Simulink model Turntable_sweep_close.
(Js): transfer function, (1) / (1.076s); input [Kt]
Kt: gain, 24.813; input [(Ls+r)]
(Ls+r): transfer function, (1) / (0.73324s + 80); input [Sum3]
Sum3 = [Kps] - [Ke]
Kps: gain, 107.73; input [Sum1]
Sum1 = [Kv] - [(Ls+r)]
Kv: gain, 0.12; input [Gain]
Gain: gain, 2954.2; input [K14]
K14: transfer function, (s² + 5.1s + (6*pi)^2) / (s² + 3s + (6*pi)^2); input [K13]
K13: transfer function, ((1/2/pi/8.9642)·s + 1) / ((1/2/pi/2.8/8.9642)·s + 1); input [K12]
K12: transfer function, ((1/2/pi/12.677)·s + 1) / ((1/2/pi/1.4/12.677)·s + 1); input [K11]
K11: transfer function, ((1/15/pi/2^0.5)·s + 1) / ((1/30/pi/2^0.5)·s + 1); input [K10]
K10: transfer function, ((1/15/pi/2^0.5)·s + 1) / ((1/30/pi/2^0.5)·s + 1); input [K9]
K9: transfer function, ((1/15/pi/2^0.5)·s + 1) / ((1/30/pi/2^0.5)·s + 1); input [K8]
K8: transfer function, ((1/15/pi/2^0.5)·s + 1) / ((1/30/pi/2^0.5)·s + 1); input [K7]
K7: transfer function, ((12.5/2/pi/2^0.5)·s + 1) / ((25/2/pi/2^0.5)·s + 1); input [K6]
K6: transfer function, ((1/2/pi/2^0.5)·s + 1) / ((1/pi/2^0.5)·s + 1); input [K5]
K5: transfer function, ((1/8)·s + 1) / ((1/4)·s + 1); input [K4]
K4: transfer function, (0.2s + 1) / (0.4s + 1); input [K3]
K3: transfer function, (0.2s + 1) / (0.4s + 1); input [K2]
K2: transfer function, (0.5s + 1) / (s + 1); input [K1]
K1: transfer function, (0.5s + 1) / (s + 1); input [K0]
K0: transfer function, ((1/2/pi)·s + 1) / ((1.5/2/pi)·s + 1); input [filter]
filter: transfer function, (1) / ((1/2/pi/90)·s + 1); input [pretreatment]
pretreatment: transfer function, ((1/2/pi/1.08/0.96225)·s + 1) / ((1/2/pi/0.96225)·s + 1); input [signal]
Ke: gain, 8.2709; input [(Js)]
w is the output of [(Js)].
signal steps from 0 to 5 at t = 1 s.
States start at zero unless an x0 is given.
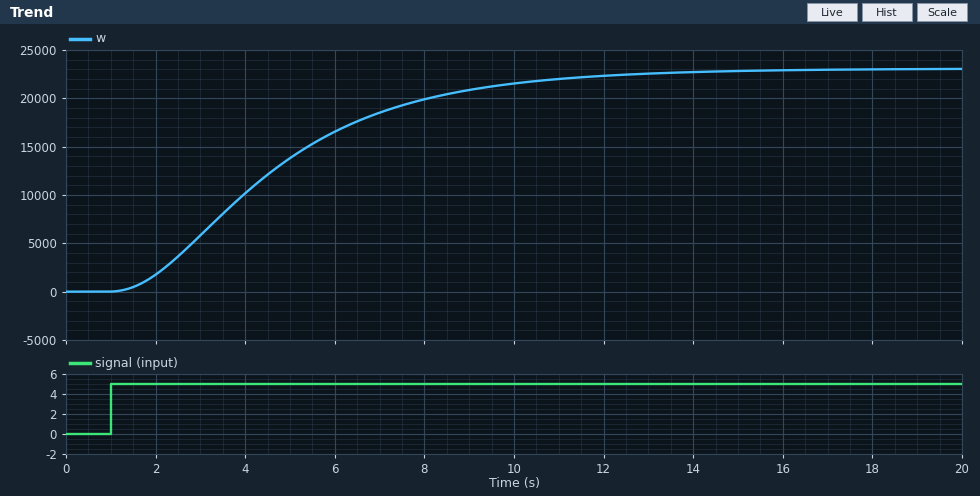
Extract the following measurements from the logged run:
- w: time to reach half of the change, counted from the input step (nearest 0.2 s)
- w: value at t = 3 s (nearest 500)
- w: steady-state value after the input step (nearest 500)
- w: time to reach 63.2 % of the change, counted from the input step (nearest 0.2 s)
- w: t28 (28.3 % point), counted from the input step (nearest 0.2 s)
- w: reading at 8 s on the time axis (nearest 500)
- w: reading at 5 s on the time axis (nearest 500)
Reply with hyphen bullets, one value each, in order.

- 3.4 s
- 6000
- 23000
- 4.2 s
- 2.2 s
- 20000
- 14000
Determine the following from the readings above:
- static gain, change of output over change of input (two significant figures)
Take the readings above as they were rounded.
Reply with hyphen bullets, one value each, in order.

- 4600
